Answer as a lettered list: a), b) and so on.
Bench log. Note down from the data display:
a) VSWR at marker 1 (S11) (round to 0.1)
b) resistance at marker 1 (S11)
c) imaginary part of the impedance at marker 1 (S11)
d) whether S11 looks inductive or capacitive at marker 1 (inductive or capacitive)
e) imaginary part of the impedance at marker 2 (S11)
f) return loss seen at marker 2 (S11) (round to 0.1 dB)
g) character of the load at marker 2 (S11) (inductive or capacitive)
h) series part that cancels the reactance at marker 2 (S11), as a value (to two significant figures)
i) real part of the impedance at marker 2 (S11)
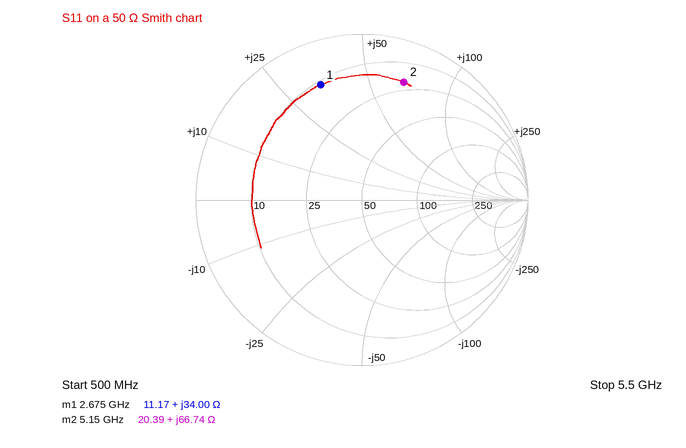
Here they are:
a) 6.6
b) 11.17 Ω
c) +34.00 Ω
d) inductive
e) +66.74 Ω
f) 2.5 dB
g) inductive
h) 460 fF
i) 20.39 Ω
